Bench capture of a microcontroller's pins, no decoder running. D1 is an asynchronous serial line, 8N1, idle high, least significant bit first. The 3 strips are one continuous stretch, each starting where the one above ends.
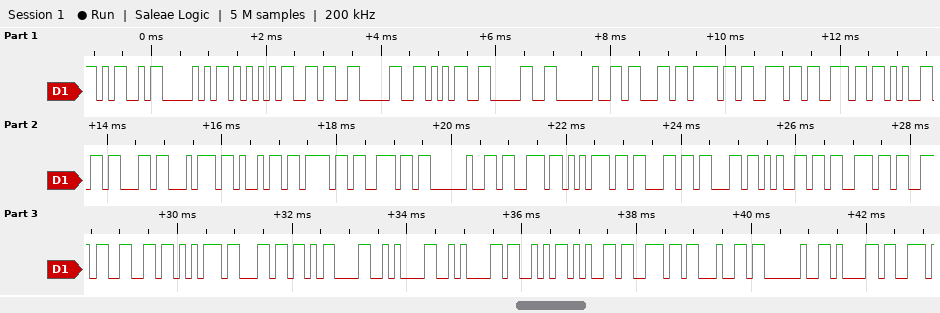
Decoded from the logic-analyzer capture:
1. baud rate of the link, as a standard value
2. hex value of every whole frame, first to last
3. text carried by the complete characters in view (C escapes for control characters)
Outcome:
9600 baud
0x4D 0x50 0x55 0x36 0x30 0x35 0x30 0x20 0x63 0x6F 0x6E 0x6E 0x65 0x63 0x74 0x69 0x6F 0x6E 0x20 0x73 0x75 0x63 0x63 0x65 0x73 0x73 0x66 0x75 0x6C 0x0D 0x0A 0x0A 0x53 0x65 0x6E 0x64 0x20 0x61
"MPU6050 connection successful\r\n\nSend a"
